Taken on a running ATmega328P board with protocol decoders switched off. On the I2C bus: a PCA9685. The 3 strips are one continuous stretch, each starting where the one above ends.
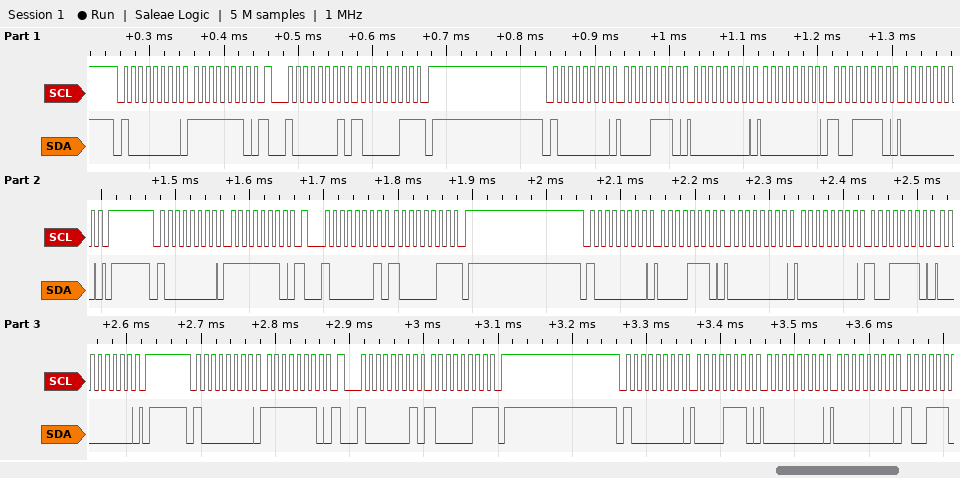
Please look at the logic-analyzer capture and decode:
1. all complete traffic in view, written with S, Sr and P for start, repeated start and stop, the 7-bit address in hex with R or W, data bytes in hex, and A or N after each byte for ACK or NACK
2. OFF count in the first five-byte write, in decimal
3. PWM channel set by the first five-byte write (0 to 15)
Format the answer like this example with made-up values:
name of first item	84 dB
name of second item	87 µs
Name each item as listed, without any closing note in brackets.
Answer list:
all complete traffic in view, written with S, Sr and P for start, repeated start and stop, the 7-bit address in hex with R or W, data bytes in hex, and A or N after each byte for ACK or NACK	S 40W A FE A Sr 40R A 83 N P S 40W A 0E A 00 A 00 A 9E A 00 A P S 40W A FE A Sr 40R A 83 N P S 40W A 0E A 00 A 00 A 9E A 00 A P S 40W A FE A Sr 40R A 83 N P S 40W A 0E A 00 A 00 A
OFF count in the first five-byte write, in decimal	158
PWM channel set by the first five-byte write	2
